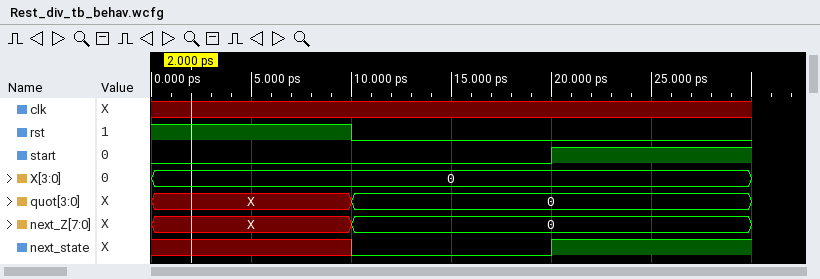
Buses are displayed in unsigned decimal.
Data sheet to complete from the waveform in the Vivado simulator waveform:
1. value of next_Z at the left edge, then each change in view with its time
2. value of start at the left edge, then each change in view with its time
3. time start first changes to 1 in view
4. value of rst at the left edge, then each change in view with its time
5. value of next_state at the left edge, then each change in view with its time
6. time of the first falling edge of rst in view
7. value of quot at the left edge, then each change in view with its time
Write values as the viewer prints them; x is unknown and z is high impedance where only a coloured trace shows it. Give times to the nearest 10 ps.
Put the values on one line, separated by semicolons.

X, 0 at 10 ps; 0, 1 at 20 ps; 20 ps; 1, 0 at 10 ps; x, 0 at 10 ps, 1 at 20 ps; 10 ps; X, 0 at 10 ps
